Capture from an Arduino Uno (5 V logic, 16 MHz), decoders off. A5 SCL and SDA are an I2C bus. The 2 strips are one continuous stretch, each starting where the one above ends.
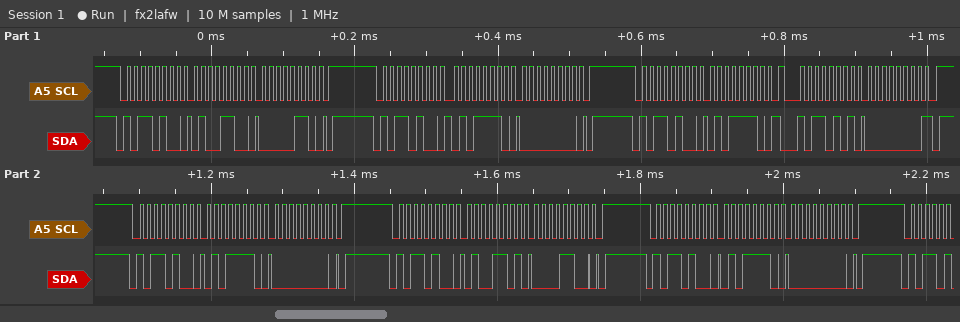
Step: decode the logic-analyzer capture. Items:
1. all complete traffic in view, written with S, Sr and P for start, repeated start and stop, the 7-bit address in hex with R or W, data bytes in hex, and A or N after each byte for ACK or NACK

S 5AW A 4C A 06 A P S 5AW A 5E A 00 A P S 5AW A 5E A Sr 5AR A 00 N P S 5AW A 5E A 00 A P S 5AW A 4D A 0C A P S 5AW A 5E A 00 A P
